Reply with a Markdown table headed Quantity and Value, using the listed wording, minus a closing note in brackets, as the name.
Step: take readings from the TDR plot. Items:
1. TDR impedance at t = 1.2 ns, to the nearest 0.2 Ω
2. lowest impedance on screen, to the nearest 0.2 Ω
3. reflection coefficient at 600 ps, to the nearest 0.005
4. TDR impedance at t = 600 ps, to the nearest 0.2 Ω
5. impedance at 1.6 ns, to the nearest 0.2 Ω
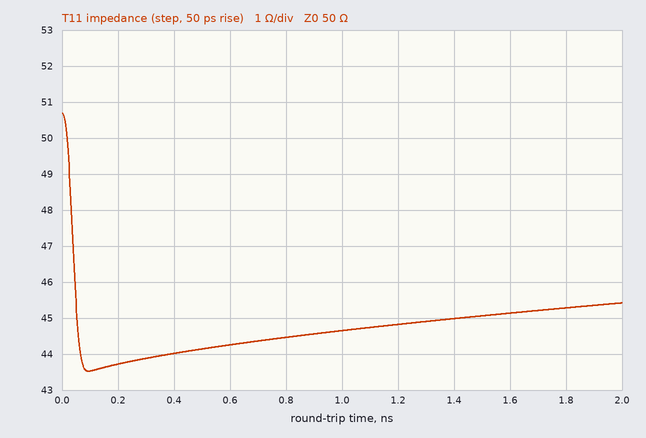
| Quantity | Value |
|---|---|
| TDR impedance at t = 1.2 ns, to the nearest 0.2 Ω | 44.8 Ω |
| lowest impedance on screen, to the nearest 0.2 Ω | 43.6 Ω |
| reflection coefficient at 600 ps, to the nearest 0.005 | -0.060 |
| TDR impedance at t = 600 ps, to the nearest 0.2 Ω | 44.2 Ω |
| impedance at 1.6 ns, to the nearest 0.2 Ω | 45.2 Ω |
